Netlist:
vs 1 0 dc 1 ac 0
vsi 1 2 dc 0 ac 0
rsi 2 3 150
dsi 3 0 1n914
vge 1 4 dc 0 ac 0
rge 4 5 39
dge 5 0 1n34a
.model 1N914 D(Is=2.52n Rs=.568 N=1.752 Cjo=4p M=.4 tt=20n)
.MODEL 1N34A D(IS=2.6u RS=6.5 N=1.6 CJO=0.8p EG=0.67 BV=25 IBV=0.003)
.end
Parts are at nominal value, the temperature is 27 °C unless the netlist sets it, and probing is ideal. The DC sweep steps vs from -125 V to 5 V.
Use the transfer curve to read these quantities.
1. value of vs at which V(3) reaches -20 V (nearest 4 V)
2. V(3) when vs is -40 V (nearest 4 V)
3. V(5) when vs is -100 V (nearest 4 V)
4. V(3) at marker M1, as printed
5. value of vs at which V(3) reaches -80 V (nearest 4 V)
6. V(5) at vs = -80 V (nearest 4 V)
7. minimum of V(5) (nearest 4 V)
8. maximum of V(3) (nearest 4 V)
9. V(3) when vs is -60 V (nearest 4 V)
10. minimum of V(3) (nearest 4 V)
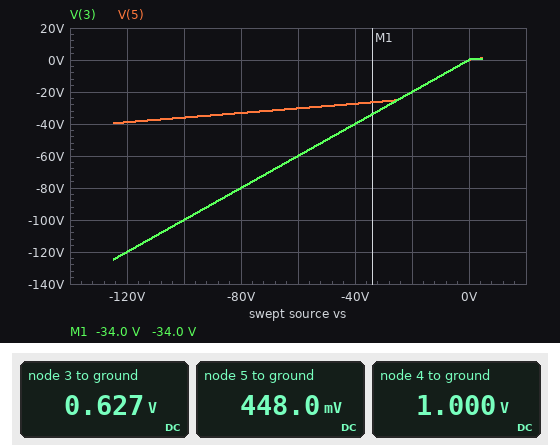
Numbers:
-20 V
-40 V
-36 V
-34.0 V
-80 V
-32 V
-40 V
0 V
-60 V
-124 V
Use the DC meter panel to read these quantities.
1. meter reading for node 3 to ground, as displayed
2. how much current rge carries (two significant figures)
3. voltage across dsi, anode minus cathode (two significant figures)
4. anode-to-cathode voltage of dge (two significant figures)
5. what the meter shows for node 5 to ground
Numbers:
0.627 V
14 mA
630 mV
450 mV
448.0 mV
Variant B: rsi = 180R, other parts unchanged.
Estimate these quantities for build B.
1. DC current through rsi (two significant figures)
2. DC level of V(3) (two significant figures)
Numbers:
2.1 mA
620 mV
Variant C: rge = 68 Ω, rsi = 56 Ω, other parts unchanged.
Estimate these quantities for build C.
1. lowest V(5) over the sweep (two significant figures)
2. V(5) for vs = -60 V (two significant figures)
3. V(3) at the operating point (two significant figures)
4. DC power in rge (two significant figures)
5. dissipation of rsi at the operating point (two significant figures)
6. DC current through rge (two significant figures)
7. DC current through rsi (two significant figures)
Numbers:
-34 V
-28 V
670 mV
5.4 mW
2.0 mW
8.9 mA
5.9 mA
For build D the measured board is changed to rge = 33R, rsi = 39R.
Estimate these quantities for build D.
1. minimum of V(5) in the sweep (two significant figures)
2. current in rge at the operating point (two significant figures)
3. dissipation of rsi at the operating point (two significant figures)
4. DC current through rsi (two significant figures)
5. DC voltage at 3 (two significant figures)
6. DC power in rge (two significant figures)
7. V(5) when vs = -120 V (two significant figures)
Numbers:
-42 V
16 mA
2.6 mW
8.1 mA
680 mV
8.6 mW
-41 V
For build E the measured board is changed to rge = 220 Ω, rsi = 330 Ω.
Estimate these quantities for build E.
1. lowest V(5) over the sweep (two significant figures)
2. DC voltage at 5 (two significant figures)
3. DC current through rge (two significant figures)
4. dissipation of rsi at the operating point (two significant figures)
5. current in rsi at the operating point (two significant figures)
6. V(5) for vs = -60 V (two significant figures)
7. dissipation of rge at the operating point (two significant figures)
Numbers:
-28 V
310 mV
3.1 mA
500 µW
1.2 mA
-26 V
2.1 mW
